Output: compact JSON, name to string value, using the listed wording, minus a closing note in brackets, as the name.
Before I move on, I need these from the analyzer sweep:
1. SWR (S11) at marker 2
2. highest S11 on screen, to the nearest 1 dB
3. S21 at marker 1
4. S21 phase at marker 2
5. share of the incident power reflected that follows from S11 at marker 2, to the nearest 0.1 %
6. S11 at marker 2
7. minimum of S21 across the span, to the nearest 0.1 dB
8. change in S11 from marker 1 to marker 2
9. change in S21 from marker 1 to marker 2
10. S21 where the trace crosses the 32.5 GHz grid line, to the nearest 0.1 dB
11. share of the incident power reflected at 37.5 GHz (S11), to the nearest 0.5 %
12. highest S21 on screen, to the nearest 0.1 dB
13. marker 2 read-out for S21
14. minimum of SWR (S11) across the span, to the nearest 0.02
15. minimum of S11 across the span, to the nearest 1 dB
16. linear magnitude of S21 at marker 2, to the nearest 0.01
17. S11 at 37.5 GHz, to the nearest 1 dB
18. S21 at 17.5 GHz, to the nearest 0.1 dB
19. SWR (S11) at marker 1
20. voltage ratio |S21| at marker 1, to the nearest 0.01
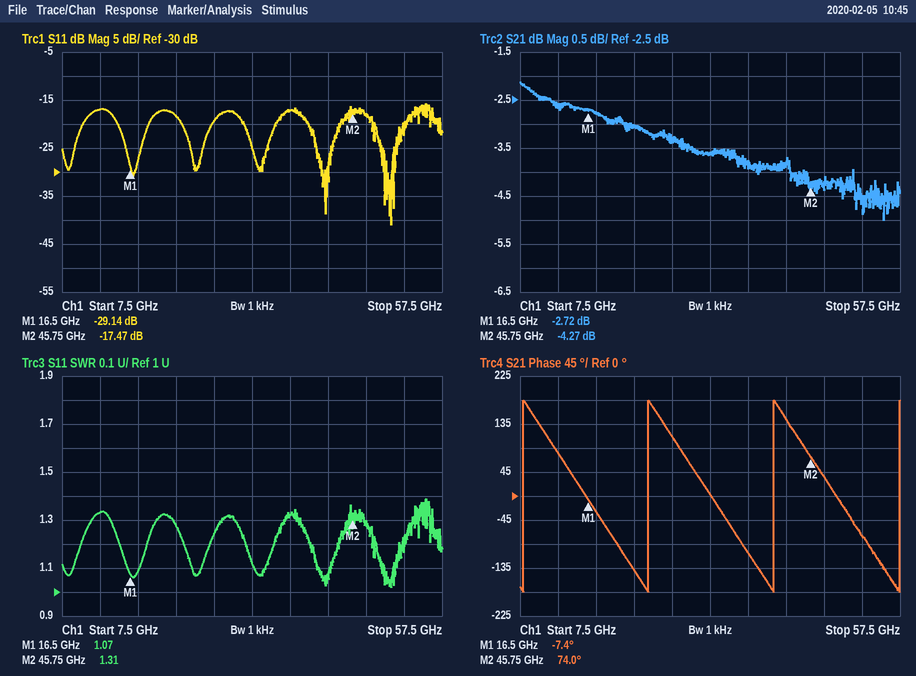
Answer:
{"SWR (S11) at marker 2": "1.31", "highest S11 on screen, to the nearest 1 dB": "-16 dB", "S21 at marker 1": "-2.72 dB", "S21 phase at marker 2": "74.0°", "share of the incident power reflected that follows from S11 at marker 2, to the nearest 0.1 %": "1.8 %", "S11 at marker 2": "-17.47 dB", "minimum of S21 across the span, to the nearest 0.1 dB": "-5.0 dB", "change in S11 from marker 1 to marker 2": "11.67 dB", "change in S21 from marker 1 to marker 2": "-1.55 dB", "S21 where the trace crosses the 32.5 GHz grid line, to the nearest 0.1 dB": "-3.6 dB", "share of the incident power reflected at 37.5 GHz (S11), to the nearest 0.5 %": "2.0 %", "highest S21 on screen, to the nearest 0.1 dB": "-2.1 dB", "marker 2 read-out for S21": "-4.27 dB", "minimum of SWR (S11) across the span, to the nearest 0.02": "1.02", "minimum of S11 across the span, to the nearest 1 dB": "-41 dB", "linear magnitude of S21 at marker 2, to the nearest 0.01": "0.61", "S11 at 37.5 GHz, to the nearest 1 dB": "-17 dB", "S21 at 17.5 GHz, to the nearest 0.1 dB": "-2.8 dB", "SWR (S11) at marker 1": "1.07", "voltage ratio |S21| at marker 1, to the nearest 0.01": "0.73"}
